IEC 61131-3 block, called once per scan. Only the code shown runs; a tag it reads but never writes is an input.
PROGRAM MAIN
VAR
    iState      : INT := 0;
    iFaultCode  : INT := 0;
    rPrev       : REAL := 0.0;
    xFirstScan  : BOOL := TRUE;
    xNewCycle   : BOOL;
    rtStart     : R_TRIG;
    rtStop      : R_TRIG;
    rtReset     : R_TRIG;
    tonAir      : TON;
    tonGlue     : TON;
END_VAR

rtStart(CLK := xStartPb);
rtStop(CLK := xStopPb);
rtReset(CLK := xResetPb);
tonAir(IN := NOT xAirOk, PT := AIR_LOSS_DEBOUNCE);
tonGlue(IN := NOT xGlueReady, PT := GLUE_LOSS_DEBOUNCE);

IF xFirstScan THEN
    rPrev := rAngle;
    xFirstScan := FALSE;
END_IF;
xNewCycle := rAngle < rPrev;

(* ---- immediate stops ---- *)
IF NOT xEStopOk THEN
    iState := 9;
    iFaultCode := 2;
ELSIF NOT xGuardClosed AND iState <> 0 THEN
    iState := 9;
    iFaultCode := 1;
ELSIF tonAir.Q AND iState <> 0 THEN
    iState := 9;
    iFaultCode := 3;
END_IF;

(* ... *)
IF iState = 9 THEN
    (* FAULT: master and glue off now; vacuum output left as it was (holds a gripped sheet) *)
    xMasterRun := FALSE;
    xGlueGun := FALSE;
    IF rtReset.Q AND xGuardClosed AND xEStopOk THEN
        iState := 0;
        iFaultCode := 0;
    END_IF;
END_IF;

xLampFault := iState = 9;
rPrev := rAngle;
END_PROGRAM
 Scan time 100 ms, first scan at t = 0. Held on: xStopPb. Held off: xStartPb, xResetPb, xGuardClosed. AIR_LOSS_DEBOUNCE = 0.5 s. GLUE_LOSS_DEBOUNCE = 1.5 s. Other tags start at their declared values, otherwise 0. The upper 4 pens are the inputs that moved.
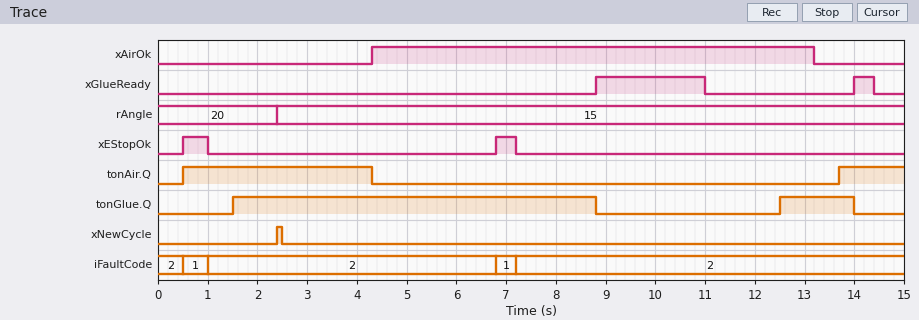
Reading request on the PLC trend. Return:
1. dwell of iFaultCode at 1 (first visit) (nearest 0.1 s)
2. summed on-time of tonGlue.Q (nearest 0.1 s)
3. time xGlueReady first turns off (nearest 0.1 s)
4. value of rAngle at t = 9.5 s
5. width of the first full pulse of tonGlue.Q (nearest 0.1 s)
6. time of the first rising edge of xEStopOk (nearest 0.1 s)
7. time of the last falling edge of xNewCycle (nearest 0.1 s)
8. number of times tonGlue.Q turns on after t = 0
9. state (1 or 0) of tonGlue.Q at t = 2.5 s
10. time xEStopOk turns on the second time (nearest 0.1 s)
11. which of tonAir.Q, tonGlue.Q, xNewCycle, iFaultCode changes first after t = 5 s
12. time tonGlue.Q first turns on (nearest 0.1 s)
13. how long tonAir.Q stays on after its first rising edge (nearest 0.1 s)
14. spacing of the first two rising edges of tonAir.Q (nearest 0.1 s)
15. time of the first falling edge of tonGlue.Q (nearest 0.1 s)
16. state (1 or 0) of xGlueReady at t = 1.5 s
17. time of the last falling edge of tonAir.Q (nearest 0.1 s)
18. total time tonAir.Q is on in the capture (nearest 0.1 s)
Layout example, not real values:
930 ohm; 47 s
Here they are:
0.5 s; 8.8 s; 11.0 s; 15; 7.3 s; 0.5 s; 2.5 s; 2; 1; 6.8 s; iFaultCode; 1.5 s; 3.8 s; 13.2 s; 8.8 s; 0; 4.3 s; 5.1 s
